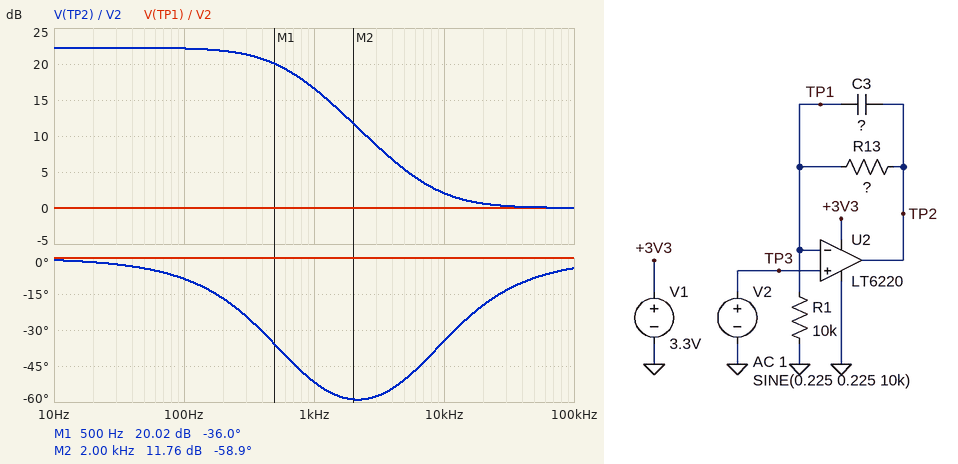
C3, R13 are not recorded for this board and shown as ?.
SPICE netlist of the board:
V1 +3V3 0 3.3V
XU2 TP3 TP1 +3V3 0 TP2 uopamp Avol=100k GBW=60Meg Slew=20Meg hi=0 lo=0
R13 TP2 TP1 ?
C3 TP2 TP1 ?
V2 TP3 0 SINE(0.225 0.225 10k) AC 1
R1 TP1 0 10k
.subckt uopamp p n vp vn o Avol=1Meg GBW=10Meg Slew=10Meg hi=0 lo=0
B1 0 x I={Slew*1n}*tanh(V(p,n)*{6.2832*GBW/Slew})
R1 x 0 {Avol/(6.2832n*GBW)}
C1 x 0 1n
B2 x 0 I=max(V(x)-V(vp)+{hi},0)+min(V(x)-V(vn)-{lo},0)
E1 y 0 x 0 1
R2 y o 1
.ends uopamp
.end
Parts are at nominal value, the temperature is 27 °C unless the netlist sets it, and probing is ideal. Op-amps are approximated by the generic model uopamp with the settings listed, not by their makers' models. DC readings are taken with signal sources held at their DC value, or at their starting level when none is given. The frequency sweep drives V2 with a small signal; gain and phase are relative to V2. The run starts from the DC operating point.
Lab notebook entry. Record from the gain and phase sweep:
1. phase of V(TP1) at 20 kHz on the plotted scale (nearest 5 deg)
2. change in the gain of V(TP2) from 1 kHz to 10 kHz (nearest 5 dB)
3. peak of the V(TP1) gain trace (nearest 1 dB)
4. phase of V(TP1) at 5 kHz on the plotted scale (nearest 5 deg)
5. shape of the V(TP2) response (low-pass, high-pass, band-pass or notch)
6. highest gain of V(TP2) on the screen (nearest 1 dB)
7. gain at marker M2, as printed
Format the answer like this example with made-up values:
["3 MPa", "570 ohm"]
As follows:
["0 deg", "-15 dB", "0 dB", "0 deg", "low-pass", "22 dB", "11.76 dB"]
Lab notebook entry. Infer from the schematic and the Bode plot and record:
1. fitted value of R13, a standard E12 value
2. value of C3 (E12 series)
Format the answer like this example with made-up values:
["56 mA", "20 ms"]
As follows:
["120 kΩ", "2.2 nF"]
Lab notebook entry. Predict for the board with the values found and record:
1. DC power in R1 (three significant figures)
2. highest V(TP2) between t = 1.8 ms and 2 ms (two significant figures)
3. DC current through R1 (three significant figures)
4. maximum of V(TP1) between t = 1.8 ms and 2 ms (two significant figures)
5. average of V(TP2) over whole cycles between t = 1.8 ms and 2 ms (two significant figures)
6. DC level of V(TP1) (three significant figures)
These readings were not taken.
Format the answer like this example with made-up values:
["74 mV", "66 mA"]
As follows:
["5.06 µW", "3.2 V", "22.5 µA", "450 mV", "2.9 V", "225 mV"]
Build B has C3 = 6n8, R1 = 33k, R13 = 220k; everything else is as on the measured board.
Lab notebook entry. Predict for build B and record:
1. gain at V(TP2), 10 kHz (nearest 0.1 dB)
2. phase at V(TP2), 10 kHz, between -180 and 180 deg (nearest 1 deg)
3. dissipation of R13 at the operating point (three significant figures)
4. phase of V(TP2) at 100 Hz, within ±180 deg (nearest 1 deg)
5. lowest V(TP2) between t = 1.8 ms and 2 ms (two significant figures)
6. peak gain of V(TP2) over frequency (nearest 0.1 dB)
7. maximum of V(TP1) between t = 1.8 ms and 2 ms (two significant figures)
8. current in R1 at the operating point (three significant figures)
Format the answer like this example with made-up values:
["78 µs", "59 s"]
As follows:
["0 dB", "-4 deg", "10.2 µW", "-36 deg", "1.5 V", "17.7 dB", "450 mV", "6.82 µA"]
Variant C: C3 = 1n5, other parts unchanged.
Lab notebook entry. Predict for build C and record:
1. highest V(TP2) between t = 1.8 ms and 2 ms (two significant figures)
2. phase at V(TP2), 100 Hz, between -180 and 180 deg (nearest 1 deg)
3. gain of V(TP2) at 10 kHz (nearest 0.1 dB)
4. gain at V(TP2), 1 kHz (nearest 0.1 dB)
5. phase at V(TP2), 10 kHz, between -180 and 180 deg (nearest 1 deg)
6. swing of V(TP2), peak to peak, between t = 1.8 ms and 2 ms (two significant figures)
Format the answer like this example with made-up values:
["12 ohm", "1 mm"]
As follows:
["3.3 V", "-6 deg", "3.6 dB", "18.7 dB", "-44 deg", "680 mV"]
